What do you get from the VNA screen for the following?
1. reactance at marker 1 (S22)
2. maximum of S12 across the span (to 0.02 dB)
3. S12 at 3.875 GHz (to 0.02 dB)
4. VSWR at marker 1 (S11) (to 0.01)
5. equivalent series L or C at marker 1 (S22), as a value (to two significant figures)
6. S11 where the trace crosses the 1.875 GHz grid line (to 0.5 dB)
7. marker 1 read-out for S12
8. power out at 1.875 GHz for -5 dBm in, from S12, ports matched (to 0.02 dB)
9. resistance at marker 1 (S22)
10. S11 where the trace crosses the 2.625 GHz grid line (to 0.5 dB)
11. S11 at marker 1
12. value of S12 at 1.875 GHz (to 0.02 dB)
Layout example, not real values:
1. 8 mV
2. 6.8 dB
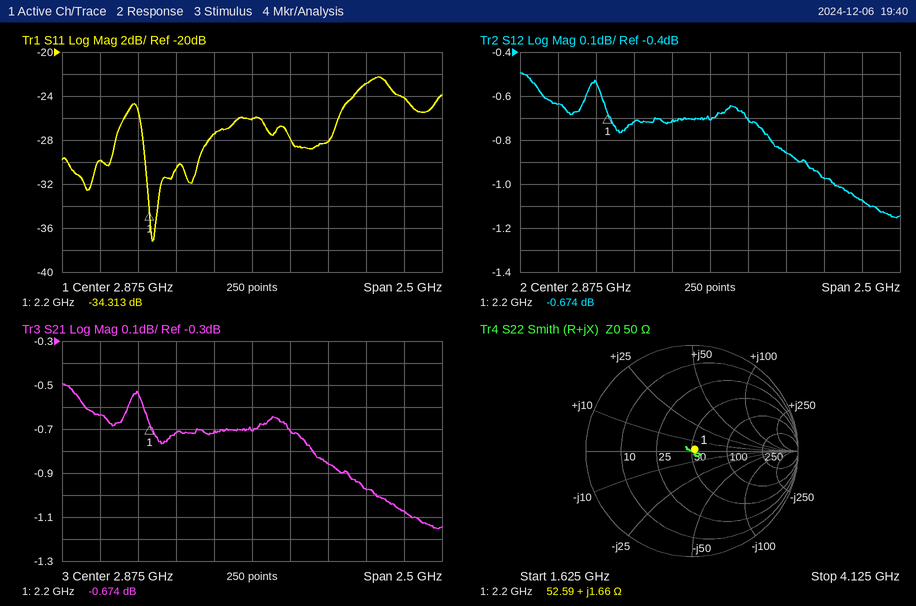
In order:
1. +1.66 Ω
2. -0.50 dB
3. -1.08 dB
4. 1.04
5. 120 pH
6. -30.0 dB
7. -0.674 dB
8. -5.64 dBm
9. 52.59 Ω
10. -27.5 dB
11. -34.313 dB
12. -0.64 dB
